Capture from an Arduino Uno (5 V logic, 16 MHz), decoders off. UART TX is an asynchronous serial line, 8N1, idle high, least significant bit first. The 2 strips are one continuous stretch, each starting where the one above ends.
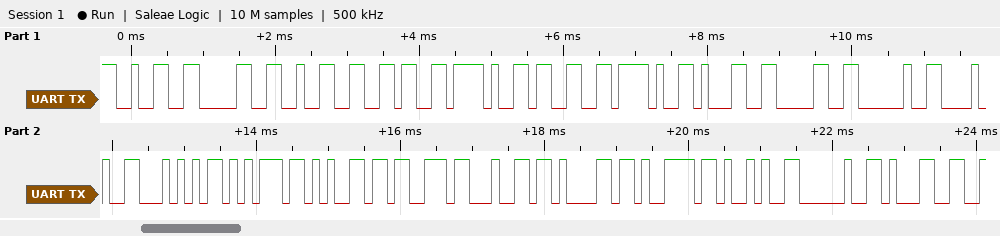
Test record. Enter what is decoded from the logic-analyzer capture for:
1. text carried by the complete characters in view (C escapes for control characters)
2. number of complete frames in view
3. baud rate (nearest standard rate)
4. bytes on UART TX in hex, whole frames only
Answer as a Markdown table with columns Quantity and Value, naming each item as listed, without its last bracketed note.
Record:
| Quantity | Value |
|---|---|
| text carried by the complete characters in view | "2026/3/10 (Tuesday) 1" |
| number of complete frames in view | 21 |
| baud rate | 9600 baud |
| bytes on UART TX in hex, whole frames only | 32 30 32 36 2F 33 2F 31 30 20 28 54 75 65 73 64 61 79 29 20 31 |
